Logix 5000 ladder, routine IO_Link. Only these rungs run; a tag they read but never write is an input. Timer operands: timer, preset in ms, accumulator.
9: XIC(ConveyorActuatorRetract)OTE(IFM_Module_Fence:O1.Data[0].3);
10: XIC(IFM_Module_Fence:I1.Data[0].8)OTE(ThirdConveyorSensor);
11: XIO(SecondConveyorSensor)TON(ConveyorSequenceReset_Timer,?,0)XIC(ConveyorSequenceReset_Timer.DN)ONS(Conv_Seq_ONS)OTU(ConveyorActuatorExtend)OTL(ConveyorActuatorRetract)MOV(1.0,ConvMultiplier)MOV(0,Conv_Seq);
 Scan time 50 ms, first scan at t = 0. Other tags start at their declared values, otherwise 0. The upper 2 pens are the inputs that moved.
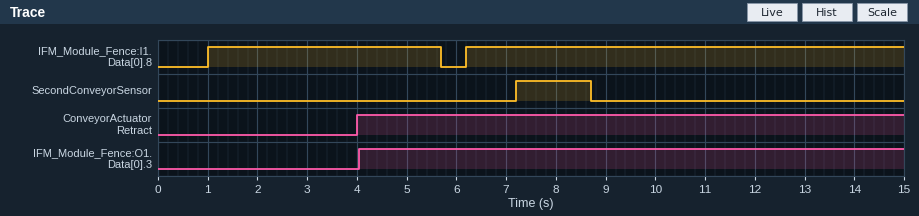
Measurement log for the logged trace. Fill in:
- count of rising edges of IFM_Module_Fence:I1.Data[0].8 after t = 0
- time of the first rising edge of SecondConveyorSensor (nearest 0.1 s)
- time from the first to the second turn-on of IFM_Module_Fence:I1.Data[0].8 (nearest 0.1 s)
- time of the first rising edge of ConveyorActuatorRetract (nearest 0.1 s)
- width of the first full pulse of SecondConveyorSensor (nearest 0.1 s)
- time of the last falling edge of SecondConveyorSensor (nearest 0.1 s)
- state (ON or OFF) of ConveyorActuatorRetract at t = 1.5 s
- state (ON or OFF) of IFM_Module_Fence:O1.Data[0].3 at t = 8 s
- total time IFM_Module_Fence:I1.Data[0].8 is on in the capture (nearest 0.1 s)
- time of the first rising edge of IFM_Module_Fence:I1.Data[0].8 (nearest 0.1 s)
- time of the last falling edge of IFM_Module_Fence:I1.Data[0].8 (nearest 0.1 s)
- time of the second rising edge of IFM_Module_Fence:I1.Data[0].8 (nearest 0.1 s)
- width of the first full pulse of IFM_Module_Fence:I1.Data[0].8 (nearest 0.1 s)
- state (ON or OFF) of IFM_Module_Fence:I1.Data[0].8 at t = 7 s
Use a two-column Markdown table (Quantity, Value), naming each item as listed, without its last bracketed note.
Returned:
| Quantity | Value |
|---|---|
| count of rising edges of IFM_Module_Fence:I1.Data[0].8 after t = 0 | 2 |
| time of the first rising edge of SecondConveyorSensor | 7.2 s |
| time from the first to the second turn-on of IFM_Module_Fence:I1.Data[0].8 | 5.2 s |
| time of the first rising edge of ConveyorActuatorRetract | 4.0 s |
| width of the first full pulse of SecondConveyorSensor | 1.5 s |
| time of the last falling edge of SecondConveyorSensor | 8.7 s |
| state (ON or OFF) of ConveyorActuatorRetract at t = 1.5 s | OFF |
| state (ON or OFF) of IFM_Module_Fence:O1.Data[0].3 at t = 8 s | ON |
| total time IFM_Module_Fence:I1.Data[0].8 is on in the capture | 13.5 s |
| time of the first rising edge of IFM_Module_Fence:I1.Data[0].8 | 1.0 s |
| time of the last falling edge of IFM_Module_Fence:I1.Data[0].8 | 5.7 s |
| time of the second rising edge of IFM_Module_Fence:I1.Data[0].8 | 6.2 s |
| width of the first full pulse of IFM_Module_Fence:I1.Data[0].8 | 4.7 s |
| state (ON or OFF) of IFM_Module_Fence:I1.Data[0].8 at t = 7 s | ON |
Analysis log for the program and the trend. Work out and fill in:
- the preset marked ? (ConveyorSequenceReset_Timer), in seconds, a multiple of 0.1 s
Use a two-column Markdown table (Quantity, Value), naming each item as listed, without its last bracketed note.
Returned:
| Quantity | Value |
|---|---|
| the preset marked ? (ConveyorSequenceReset_Timer), in seconds, a multiple of 0.1 s | 4.0 s |
